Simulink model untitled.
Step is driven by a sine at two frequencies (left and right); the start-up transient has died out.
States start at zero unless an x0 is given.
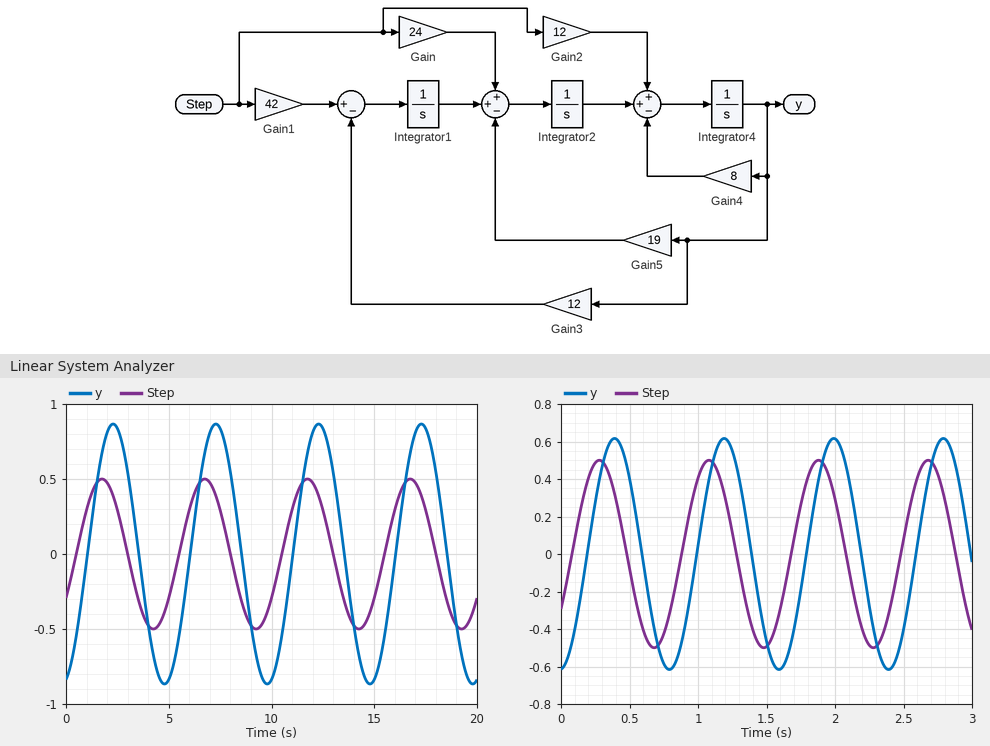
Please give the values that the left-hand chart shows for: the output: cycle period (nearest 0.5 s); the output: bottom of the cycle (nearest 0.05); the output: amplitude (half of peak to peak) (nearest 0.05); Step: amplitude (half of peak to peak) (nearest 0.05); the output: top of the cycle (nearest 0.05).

5.0 s
-0.85
0.85
0.50
0.85
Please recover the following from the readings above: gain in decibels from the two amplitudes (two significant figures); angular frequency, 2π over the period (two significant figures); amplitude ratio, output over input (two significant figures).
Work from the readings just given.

4.6 dB
1.3 rad/s
1.7
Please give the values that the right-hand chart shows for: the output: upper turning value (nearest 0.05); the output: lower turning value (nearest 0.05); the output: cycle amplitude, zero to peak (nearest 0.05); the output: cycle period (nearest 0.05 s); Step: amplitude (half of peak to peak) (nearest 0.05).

0.60
-0.60
0.60
0.80 s
0.50
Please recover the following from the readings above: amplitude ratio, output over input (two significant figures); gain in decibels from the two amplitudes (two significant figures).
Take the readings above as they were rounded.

1.2
1.6 dB
